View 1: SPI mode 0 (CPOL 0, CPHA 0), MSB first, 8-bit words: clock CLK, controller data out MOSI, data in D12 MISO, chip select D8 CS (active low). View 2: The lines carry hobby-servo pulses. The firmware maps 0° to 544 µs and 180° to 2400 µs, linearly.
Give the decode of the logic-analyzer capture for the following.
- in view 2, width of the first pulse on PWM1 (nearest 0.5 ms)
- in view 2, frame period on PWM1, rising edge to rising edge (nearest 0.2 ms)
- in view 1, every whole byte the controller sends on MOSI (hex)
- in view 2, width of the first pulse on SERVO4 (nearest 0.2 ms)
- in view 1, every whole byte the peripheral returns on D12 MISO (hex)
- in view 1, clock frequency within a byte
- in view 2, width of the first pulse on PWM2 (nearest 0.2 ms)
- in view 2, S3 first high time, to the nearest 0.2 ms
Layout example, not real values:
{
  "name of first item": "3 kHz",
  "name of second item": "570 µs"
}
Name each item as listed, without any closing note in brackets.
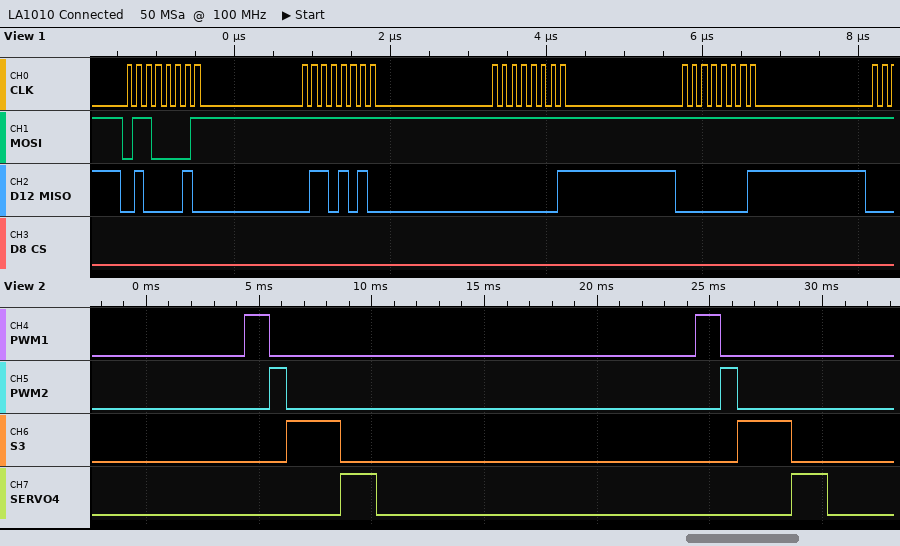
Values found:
{
  "in view 2, width of the first pulse on PWM1": "1.0 ms",
  "in view 2, frame period on PWM1, rising edge to rising edge": "20.0 ms",
  "in view 1, every whole byte the controller sends on MOSI": "61 FF FF FF",
  "in view 2, width of the first pulse on SERVO4": "1.6 ms",
  "in view 1, every whole byte the peripheral returns on D12 MISO": "42 6A 01 01",
  "in view 1, clock frequency within a byte": "8 MHz",
  "in view 2, width of the first pulse on PWM2": "0.8 ms",
  "in view 2, S3 first high time, to the nearest 0.2 ms": "2.4 ms"
}
